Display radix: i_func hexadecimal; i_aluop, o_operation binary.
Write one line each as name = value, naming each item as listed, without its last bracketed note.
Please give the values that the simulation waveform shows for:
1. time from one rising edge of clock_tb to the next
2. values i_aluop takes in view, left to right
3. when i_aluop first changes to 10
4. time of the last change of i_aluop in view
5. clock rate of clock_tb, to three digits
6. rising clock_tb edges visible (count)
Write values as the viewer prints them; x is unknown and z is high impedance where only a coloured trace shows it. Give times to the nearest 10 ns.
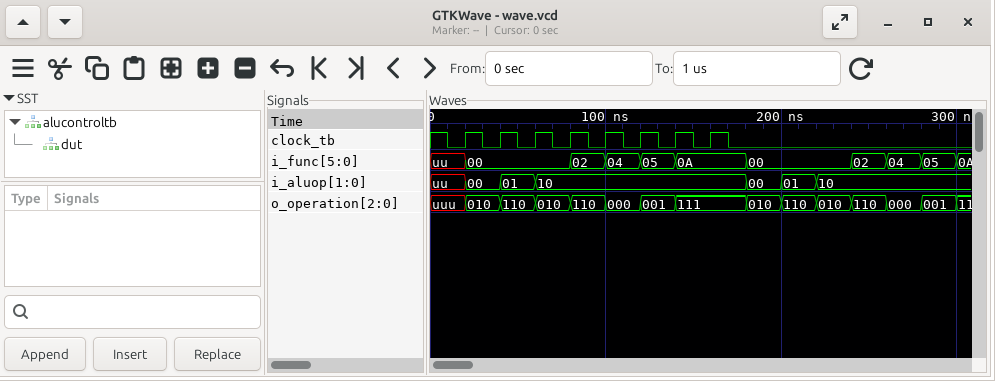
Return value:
time from one rising edge of clock_tb to the next = 20 ns
values i_aluop takes in view, left to right = uu, 00, 01, 10, 00, 01, 10
when i_aluop first changes to 10 = 60 ns
time of the last change of i_aluop in view = 220 ns
clock rate of clock_tb, to three digits = 50.0 MHz
rising clock_tb edges visible = 8
